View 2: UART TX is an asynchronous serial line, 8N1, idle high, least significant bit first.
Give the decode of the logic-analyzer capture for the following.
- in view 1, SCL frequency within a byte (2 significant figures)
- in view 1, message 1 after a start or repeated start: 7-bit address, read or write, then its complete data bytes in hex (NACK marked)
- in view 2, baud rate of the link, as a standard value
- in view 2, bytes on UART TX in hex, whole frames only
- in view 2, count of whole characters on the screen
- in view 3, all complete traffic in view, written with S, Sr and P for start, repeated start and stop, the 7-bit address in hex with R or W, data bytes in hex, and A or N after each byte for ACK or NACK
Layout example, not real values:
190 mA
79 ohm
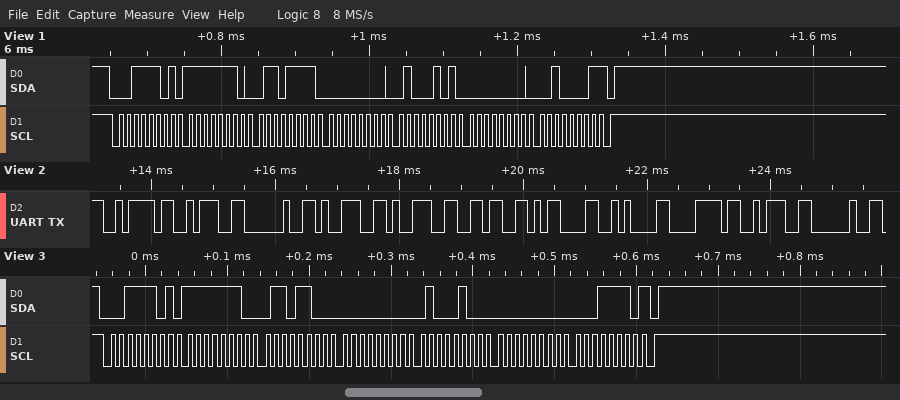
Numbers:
100 kHz
0x1E read: FE 6F 00 45 00 21 NACK
9600 baud
7A 3A 20 39 39 36 0D 0A 78 3A 20
11
S 1ER A FE A 6C A 00 A 44 A 00 A 1E N P
